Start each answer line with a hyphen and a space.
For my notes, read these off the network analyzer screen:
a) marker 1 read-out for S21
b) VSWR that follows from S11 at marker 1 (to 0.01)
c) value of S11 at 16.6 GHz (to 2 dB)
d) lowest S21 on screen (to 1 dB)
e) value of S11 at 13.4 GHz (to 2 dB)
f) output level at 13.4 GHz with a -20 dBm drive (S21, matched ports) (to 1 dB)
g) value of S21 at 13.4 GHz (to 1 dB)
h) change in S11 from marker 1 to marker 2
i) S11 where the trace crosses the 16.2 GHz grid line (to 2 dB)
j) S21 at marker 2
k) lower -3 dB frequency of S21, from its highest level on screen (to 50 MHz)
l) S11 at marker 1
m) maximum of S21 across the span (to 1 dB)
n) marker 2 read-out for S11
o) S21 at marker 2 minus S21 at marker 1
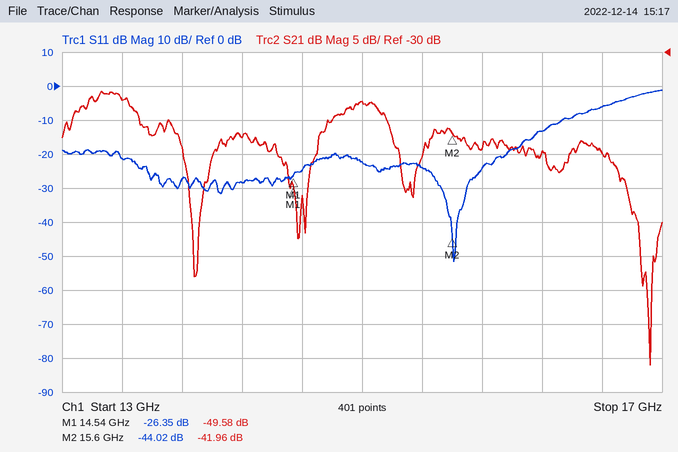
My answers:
- -49.58 dB
- 1.10
- -6 dB
- -76 dB
- -22 dB
- -57 dBm
- -37 dB
- -17.67 dB
- -14 dB
- -41.96 dB
- 13.10 GHz
- -26.35 dB
- -36 dB
- -44.02 dB
- 7.62 dB
